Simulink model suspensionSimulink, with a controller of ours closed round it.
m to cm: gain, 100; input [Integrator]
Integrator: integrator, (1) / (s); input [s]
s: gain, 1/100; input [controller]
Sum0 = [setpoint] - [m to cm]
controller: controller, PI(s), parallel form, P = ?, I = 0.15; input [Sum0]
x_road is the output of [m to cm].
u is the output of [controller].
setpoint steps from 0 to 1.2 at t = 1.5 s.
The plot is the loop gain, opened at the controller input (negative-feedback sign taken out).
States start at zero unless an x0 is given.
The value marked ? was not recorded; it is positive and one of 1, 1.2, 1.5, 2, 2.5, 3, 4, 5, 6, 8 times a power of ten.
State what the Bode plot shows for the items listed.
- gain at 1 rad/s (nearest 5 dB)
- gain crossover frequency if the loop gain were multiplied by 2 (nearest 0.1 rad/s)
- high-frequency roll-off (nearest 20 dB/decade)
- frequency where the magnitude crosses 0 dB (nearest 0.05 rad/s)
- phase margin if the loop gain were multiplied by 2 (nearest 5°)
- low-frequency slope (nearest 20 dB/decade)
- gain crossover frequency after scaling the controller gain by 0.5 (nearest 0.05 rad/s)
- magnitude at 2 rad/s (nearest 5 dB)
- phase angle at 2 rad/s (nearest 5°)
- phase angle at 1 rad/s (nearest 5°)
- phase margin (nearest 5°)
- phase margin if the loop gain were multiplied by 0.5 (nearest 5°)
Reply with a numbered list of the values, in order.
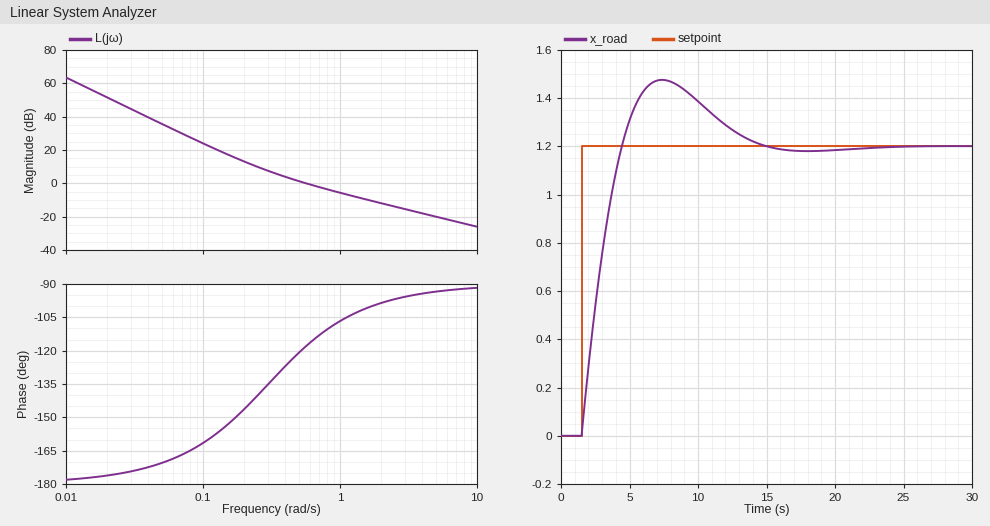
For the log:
1. -5 dB
2. 1.0 rad/s
3. -20 dB/decade
4. 0.55 rad/s
5. 75°
6. -40 dB/decade
7. 0.35 rad/s
8. -10 dB
9. -100°
10. -105°
11. 60°
12. 50°
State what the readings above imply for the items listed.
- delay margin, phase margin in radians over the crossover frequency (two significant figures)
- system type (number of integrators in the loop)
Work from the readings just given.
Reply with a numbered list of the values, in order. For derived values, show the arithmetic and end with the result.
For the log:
1. 60 × π / 180 / 0.55 = 1.9 s
2. 2
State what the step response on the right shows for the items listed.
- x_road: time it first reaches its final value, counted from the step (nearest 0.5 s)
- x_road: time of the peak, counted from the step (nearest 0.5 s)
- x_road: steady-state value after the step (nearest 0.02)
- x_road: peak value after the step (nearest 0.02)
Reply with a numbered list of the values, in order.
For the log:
1. 3.0 s
2. 6.0 s
3. 1.20
4. 1.48
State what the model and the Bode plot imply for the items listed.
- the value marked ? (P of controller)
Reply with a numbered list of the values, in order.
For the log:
1. 0.5
